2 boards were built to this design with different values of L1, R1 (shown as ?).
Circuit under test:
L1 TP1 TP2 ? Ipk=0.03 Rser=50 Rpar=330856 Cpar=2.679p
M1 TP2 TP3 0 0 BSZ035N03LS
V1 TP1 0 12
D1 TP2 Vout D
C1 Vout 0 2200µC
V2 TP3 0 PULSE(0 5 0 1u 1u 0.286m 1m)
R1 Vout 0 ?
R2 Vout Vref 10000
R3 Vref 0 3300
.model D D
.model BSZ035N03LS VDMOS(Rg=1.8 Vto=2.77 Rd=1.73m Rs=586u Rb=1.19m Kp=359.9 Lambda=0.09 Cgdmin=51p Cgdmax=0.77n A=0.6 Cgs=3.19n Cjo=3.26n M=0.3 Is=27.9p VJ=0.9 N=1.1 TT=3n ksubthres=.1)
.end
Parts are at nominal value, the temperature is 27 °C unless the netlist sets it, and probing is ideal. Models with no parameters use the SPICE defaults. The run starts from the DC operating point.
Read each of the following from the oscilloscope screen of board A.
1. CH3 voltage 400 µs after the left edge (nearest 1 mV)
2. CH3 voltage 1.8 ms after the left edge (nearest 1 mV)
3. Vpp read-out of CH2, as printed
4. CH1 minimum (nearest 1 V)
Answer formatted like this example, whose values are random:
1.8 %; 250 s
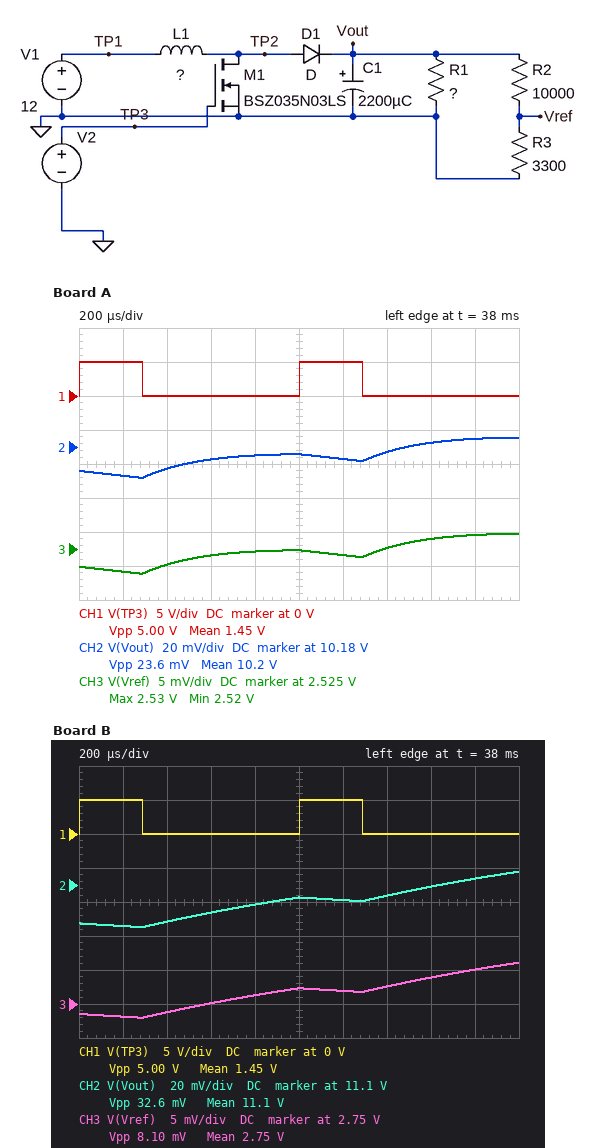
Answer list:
2.523 V; 2.527 V; 23.6 mV; 0 V
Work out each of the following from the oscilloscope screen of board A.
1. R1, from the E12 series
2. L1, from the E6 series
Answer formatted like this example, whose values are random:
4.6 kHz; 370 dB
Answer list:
330 Ω; 15 mH
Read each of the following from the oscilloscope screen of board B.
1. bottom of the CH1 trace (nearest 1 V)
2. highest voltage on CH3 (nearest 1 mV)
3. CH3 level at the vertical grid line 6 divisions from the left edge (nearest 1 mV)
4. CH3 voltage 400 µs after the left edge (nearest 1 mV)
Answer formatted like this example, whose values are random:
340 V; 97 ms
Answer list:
0 V; 2.756 V; 2.752 V; 2.749 V
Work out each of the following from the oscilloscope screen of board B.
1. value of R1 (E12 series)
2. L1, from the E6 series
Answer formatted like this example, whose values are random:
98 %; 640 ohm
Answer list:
680 Ω; 100 mH
